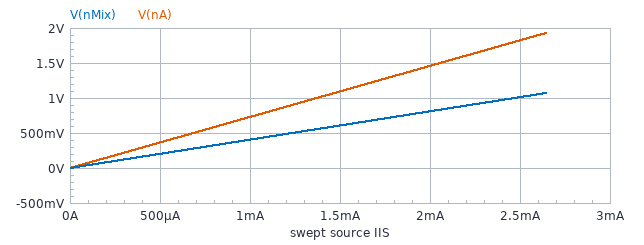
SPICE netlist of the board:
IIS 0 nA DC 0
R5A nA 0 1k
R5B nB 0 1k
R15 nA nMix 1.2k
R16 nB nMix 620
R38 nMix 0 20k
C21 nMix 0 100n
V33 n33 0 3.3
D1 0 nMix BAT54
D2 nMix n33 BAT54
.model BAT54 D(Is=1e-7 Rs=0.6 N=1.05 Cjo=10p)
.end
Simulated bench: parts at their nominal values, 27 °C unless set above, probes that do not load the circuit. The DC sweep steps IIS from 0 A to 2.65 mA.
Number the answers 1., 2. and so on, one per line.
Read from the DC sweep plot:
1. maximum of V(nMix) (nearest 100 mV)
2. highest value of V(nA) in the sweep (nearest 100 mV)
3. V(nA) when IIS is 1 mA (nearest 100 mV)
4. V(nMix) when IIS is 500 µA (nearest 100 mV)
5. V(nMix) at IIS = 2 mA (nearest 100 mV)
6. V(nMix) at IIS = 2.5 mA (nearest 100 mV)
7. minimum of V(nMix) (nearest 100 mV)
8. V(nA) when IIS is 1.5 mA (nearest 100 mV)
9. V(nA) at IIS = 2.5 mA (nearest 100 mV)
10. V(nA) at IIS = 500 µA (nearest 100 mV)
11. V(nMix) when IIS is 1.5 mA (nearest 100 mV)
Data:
1. 1.1 V
2. 1.9 V
3. 700 mV
4. 200 mV
5. 800 mV
6. 1.0 V
7. 0 V
8. 1.1 V
9. 1.8 V
10. 400 mV
11. 600 mV
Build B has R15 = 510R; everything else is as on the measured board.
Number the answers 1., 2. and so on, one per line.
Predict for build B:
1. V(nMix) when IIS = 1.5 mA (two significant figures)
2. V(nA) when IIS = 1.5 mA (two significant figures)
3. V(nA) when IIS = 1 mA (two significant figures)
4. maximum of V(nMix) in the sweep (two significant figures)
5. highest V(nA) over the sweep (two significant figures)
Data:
1. 750 mV
2. 1.0 V
3. 670 mV
4. 1.3 V
5. 1.8 V
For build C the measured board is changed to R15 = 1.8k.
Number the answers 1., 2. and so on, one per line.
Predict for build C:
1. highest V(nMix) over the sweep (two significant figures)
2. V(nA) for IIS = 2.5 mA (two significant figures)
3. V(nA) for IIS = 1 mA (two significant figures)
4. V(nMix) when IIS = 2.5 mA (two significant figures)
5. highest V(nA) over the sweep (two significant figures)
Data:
1. 920 mV
2. 1.9 V
3. 770 mV
4. 870 mV
5. 2.0 V
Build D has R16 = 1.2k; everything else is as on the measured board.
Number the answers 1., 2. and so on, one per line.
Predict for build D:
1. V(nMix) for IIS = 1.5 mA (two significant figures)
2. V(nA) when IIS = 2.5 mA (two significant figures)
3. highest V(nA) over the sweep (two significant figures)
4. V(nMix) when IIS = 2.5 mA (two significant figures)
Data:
1. 710 mV
2. 1.9 V
3. 2.0 V
4. 1.2 V
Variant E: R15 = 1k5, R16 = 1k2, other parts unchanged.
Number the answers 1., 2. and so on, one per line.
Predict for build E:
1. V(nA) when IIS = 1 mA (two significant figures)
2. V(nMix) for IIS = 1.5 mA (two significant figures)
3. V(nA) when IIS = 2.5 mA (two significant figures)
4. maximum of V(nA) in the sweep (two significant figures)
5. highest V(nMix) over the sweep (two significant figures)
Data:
1. 780 mV
2. 660 mV
3. 1.9 V
4. 2.1 V
5. 1.2 V
